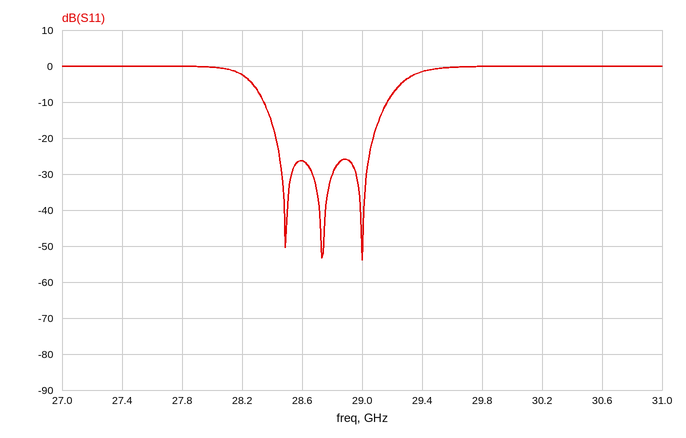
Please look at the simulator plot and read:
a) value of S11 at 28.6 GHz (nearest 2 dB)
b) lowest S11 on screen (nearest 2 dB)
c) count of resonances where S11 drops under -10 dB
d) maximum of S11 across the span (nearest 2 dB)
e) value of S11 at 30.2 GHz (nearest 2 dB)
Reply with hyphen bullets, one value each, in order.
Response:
- -26 dB
- -54 dB
- 3
- 0 dB
- 0 dB
